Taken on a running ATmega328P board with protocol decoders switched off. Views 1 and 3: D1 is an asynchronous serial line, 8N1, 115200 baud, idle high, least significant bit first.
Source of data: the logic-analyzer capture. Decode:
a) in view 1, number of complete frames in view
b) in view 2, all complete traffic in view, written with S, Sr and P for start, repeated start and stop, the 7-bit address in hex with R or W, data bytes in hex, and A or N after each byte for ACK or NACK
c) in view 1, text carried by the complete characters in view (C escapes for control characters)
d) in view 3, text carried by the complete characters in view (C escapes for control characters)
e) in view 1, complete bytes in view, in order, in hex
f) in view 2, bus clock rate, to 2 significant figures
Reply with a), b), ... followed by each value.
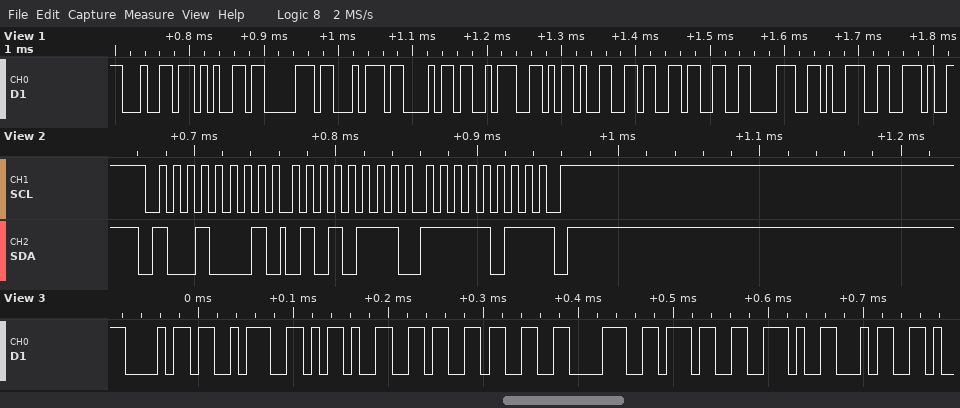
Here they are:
a) 12
b) S 48R A 57 A FB N P
c) "depth:-6389."
d) "h:-6387.4"
e) 0x64 0x65 0x70 0x74 0x68 0x3A 0x2D 0x36 0x33 0x38 0x39 0x2E
f) 100 kHz
